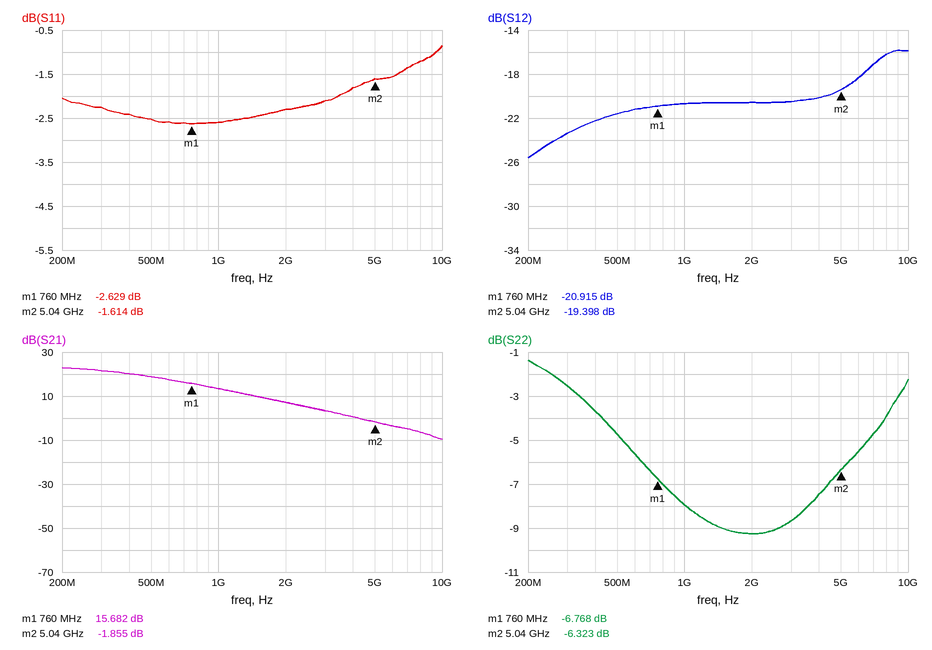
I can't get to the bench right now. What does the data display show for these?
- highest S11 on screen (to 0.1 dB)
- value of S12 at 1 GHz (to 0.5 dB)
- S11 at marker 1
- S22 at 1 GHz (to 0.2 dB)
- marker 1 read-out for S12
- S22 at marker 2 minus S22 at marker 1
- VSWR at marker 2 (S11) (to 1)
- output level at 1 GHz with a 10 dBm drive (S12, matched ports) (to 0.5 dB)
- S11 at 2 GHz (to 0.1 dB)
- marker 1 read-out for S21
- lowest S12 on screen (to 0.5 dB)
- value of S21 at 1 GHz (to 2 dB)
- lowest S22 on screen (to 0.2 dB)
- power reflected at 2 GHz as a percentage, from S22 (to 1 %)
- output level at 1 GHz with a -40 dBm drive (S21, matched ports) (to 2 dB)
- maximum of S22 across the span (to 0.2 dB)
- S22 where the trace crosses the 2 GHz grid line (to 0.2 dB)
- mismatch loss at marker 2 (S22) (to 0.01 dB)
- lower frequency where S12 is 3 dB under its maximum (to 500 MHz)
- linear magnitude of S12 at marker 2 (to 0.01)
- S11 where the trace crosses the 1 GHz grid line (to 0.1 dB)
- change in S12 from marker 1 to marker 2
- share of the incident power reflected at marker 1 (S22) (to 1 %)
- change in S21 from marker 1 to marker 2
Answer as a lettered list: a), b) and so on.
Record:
a) -0.9 dB
b) -20.5 dB
c) -2.629 dB
d) -8.0 dB
e) -20.915 dB
f) 0.445 dB
g) 11
h) -10.5 dBm
i) -2.3 dB
j) 15.682 dB
k) -25.5 dB
l) 14 dB
m) -9.2 dB
n) 12 %
o) -26 dBm
p) -1.4 dB
q) -9.2 dB
r) 1.15 dB
s) 5.5 GHz
t) 0.11
u) -2.6 dB
v) 1.517 dB
w) 21 %
x) -17.537 dB
